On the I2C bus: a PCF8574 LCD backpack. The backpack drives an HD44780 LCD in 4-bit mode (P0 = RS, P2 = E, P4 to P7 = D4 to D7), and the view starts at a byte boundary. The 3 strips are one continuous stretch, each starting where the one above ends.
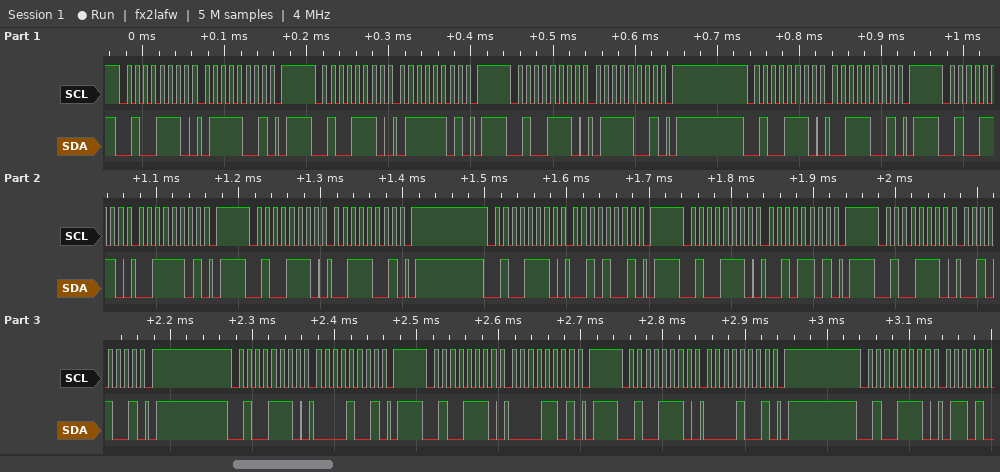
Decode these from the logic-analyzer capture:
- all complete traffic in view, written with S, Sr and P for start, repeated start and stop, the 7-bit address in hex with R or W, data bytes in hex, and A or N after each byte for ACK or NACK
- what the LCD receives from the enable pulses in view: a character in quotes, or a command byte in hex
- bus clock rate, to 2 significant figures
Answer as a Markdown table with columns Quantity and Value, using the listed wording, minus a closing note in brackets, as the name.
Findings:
| Quantity | Value |
|---|---|
| all complete traffic in view, written with S, Sr and P for start, repeated start and stop, the 7-bit address in hex with R or W, data bytes in hex, and A or N after each byte for ACK or NACK | S 27W A 79 A P S 27W A 7D A P S 27W A 79 A P S 27W A 39 A P S 27W A 3D A P S 27W A 39 A P S 27W A 29 A P S 27W A 2D A P S 27W A 29 A P S 27W A 09 A P S 27W A 0D A P S 27W A 09 A P S 27W A |
| what the LCD receives from the enable pulses in view: a character in quotes, or a command byte in hex | 's' ' ' |
| bus clock rate, to 2 significant figures | 100 kHz |
